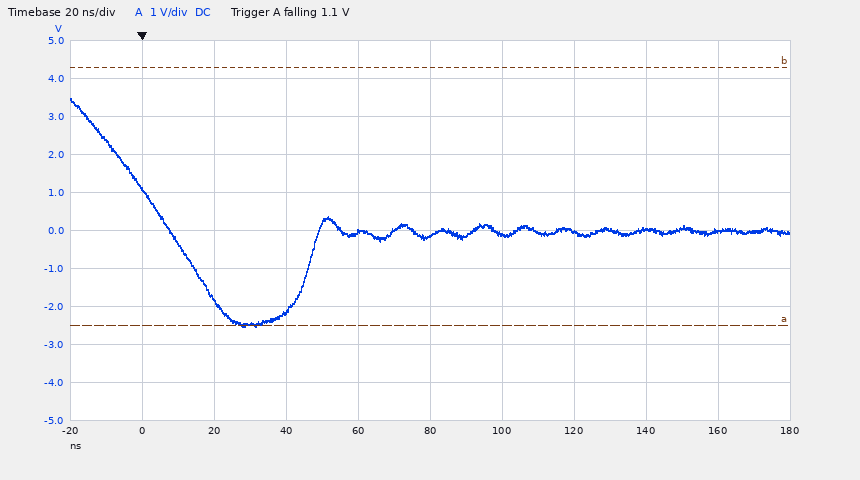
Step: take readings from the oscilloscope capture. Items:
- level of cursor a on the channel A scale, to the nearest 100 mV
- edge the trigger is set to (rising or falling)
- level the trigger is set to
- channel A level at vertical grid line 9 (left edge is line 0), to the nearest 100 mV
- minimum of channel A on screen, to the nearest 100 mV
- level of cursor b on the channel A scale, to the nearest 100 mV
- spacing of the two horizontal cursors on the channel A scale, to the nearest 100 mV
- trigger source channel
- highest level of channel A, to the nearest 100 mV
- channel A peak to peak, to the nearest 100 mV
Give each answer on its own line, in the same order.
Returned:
-2.5 V
falling
1.1 V
0.0 V
-2.5 V
4.3 V
6.8 V
channel A
3.5 V
6.0 V
